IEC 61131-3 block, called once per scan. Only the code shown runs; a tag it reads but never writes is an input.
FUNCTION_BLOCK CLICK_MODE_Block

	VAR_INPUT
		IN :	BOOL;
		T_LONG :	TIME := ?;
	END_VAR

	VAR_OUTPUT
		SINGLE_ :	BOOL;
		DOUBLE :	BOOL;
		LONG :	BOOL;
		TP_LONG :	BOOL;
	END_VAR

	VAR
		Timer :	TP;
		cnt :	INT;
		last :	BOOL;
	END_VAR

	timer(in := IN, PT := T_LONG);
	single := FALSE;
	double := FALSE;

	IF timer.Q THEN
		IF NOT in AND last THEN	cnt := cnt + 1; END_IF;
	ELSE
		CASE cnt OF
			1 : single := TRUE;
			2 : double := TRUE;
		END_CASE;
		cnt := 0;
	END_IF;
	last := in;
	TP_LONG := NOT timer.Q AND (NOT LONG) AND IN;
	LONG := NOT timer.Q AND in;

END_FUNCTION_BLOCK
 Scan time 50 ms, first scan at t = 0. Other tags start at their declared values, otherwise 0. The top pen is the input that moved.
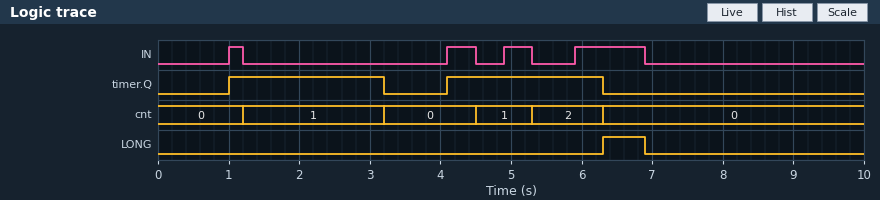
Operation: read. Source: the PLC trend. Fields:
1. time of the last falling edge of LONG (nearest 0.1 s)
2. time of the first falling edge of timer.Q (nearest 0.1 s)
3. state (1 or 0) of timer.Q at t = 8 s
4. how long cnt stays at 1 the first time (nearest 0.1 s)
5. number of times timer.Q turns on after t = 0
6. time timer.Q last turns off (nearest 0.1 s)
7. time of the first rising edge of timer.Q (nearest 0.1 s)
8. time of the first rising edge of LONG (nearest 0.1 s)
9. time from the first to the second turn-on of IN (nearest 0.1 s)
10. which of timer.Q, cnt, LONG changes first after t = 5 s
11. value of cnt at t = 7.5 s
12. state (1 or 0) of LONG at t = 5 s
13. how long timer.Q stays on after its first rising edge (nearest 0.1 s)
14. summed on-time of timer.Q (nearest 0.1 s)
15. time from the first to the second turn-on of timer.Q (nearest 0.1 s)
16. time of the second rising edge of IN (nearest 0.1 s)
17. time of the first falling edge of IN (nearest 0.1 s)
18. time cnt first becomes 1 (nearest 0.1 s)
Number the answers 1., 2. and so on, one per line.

1. 6.9 s
2. 3.2 s
3. 0
4. 2.0 s
5. 2
6. 6.3 s
7. 1.0 s
8. 6.3 s
9. 3.1 s
10. cnt
11. 0
12. 0
13. 2.2 s
14. 4.4 s
15. 3.1 s
16. 4.1 s
17. 1.2 s
18. 1.2 s
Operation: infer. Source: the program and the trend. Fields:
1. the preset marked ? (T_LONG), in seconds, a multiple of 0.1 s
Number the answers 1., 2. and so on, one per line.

1. 2.2 s
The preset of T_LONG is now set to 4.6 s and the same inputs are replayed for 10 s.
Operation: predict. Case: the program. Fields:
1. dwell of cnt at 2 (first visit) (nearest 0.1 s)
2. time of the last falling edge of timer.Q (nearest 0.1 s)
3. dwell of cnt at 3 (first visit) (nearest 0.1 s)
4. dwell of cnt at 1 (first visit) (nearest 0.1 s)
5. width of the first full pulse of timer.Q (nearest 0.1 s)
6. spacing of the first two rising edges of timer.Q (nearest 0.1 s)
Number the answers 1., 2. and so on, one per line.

1. 0.8 s
2. 5.6 s
3. 0.3 s
4. 3.3 s
5. 4.6 s
6. 4.9 s
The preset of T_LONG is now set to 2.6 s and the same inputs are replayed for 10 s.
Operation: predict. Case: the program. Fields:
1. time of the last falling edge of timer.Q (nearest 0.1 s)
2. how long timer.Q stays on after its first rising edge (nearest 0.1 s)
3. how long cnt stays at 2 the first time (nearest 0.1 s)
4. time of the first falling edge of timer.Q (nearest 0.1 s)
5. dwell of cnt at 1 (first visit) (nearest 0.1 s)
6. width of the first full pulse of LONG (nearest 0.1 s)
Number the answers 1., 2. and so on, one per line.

1. 6.7 s
2. 2.6 s
3. 1.4 s
4. 3.6 s
5. 2.4 s
6. 0.2 s
